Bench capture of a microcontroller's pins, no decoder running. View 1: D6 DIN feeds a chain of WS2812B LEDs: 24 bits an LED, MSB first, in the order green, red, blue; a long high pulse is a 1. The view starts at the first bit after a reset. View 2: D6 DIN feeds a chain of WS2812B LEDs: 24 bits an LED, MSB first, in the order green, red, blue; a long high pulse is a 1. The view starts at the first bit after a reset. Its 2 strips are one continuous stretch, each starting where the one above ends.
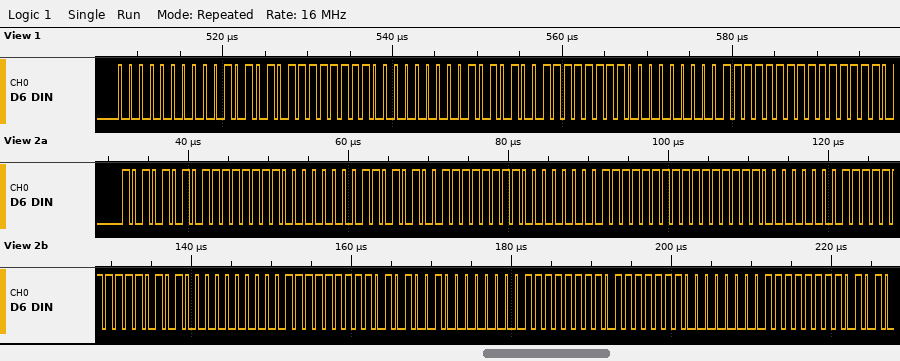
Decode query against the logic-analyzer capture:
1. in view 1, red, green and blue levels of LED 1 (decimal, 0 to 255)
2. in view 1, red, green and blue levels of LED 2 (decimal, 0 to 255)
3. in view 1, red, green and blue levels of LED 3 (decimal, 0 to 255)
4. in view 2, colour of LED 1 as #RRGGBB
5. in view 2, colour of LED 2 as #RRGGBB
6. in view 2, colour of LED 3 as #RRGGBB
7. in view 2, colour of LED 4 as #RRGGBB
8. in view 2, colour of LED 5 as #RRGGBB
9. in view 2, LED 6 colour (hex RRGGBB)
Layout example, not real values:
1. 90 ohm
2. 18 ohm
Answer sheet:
1. 42, 0, 255
2. 84, 0, 255
3. 127, 0, 255
4. #FFAA00
5. #FFD400
6. #FFFF00
7. #D4FF00
8. #A9FF00
9. #7FFF00
